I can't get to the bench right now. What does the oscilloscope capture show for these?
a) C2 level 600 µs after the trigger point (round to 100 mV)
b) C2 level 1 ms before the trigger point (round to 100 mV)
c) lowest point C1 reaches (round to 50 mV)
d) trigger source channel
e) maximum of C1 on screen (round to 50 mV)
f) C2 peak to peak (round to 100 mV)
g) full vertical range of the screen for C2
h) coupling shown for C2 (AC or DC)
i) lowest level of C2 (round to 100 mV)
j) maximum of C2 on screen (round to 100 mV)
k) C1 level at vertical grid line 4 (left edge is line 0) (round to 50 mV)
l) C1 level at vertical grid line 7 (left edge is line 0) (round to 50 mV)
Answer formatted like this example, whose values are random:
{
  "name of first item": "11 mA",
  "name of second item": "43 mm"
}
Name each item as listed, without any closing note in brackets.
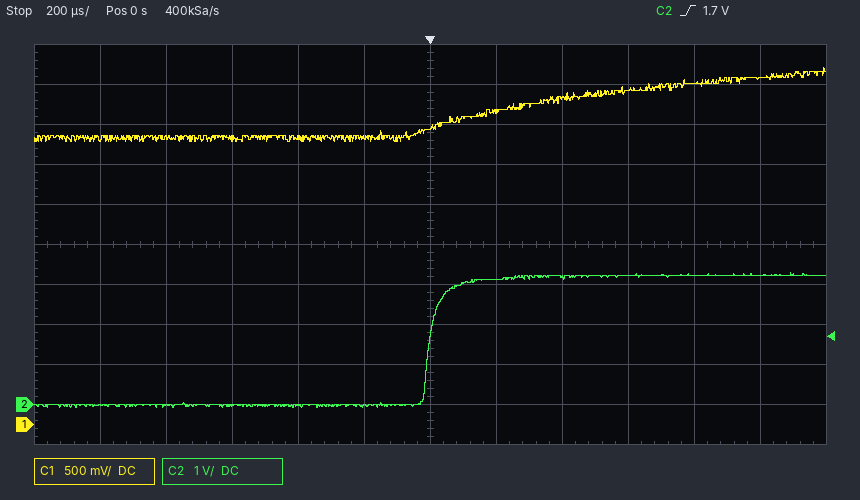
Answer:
{
  "C2 level 600 µs after the trigger point": "3.2 V",
  "C2 level 1 ms before the trigger point": "0.0 V",
  "lowest point C1 reaches": "3.55 V",
  "trigger source channel": "C2",
  "maximum of C1 on screen": "4.45 V",
  "C2 peak to peak": "3.4 V",
  "full vertical range of the screen for C2": "10 V",
  "coupling shown for C2": "DC",
  "lowest level of C2": "-100 mV",
  "maximum of C2 on screen": "3.3 V",
  "C1 level at vertical grid line 4 (left edge is line 0)": "3.60 V",
  "C1 level at vertical grid line 7 (left edge is line 0)": "3.90 V"
}
